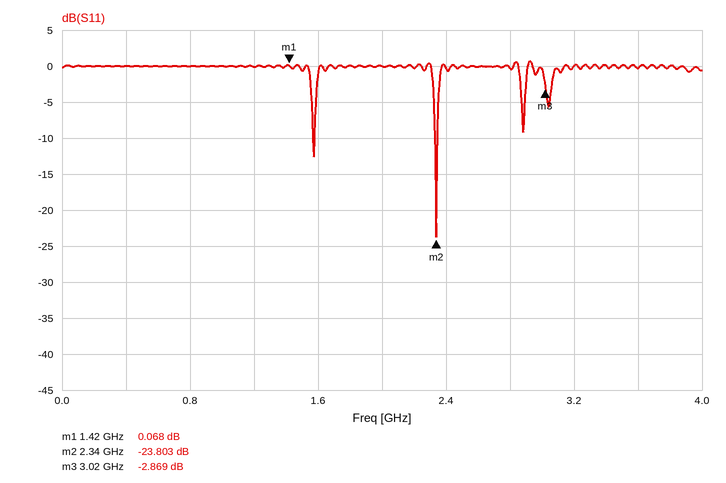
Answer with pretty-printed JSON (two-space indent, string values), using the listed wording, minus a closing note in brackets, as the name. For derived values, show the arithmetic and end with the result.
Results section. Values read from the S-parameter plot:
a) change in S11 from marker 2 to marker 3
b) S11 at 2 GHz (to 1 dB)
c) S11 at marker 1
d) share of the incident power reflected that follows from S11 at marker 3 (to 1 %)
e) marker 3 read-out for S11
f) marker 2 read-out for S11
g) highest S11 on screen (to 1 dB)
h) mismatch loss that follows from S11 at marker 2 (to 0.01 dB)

{
  "change in S11 from marker 2 to marker 3": "-2.869 − (-23.803) = 20.934 dB",
  "S11 at 2 GHz": "0 dB",
  "S11 at marker 1": "0.068 dB",
  "share of the incident power reflected that follows from S11 at marker 3": "10^(-2.869/10) ≈ 52 %",
  "marker 3 read-out for S11": "-2.869 dB",
  "marker 2 read-out for S11": "-23.803 dB",
  "highest S11 on screen": "1 dB",
  "mismatch loss that follows from S11 at marker 2": "−10 log10(1 − 10^(-23.803/10)) ≈ 0.02 dB"
}
